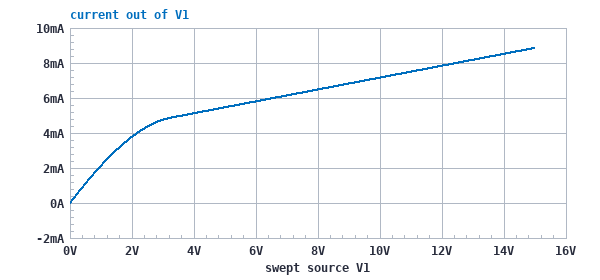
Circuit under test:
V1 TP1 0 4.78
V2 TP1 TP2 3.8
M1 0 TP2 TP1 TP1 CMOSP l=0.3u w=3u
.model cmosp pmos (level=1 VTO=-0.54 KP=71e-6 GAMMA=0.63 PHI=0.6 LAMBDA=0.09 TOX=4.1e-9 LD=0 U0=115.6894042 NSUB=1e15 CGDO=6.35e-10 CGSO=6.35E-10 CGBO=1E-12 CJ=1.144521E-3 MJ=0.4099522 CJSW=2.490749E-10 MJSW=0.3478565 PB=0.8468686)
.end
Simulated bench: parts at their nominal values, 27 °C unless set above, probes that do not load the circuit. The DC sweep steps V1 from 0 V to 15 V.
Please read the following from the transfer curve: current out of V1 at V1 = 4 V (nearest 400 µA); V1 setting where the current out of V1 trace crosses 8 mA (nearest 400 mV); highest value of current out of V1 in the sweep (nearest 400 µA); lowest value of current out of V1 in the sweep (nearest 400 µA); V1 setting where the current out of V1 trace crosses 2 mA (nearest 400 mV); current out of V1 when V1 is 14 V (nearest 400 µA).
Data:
5.2 mA
12.4 V
8.8 mA
0 A
800 mV
8.4 mA
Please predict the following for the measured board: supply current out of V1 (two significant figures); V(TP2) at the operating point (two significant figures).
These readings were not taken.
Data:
5.4 mA
980 mV
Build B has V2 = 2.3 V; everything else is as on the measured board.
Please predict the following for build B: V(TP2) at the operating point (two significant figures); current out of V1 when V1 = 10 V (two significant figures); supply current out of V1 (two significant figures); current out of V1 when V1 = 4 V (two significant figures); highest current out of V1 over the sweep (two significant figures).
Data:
2.5 V
2.1 mA
1.6 mA
1.5 mA
2.6 mA
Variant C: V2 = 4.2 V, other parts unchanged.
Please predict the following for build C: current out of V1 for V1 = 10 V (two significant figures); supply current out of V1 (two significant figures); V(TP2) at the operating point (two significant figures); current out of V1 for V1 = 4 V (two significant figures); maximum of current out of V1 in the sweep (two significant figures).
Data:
9.0 mA
6.8 mA
580 mV
6.5 mA
11 mA
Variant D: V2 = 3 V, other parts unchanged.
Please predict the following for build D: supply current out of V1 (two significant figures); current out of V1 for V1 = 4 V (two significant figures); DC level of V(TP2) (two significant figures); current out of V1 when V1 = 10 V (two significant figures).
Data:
3.1 mA
2.9 mA
1.8 V
4.1 mA
